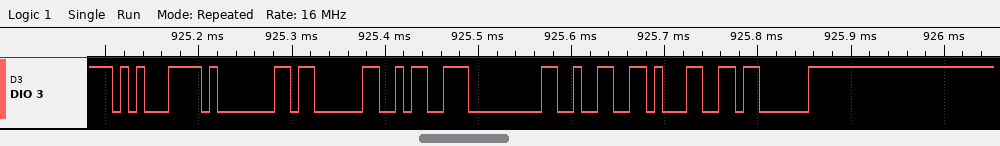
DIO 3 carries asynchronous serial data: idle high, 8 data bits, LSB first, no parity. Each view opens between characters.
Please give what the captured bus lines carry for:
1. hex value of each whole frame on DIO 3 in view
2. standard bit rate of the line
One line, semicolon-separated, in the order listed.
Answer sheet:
C5, 01, 03, 9A, 00, 32, 31, 03; 115200 baud
